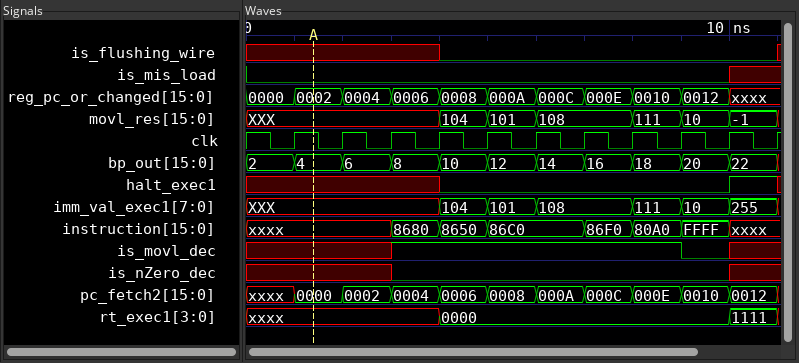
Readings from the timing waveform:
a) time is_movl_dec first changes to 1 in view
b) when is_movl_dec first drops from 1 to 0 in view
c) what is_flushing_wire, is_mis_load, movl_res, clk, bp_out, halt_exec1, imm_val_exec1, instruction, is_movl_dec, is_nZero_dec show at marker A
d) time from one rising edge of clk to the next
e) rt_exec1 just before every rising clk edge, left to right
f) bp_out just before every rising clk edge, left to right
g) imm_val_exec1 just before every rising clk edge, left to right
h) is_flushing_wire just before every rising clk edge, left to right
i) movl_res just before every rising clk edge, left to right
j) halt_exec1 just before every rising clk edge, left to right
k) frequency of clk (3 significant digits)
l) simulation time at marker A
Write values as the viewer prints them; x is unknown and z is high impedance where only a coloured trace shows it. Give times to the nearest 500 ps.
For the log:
3000 ps
9000 ps
is_flushing_wire=x, is_mis_load=0, movl_res=XXX, clk=1, bp_out=4, halt_exec1=x, imm_val_exec1=XXX, instruction=xxxx, is_movl_dec=x, is_nZero_dec=x
1000 ps
xxxx, xxxx, xxxx, xxxx, 0000, 0000, 0000, 0000, 0000, 0000, 1111
2, 4, 6, 8, 10, 12, 14, 16, 18, 20, 22
XXX, XXX, XXX, XXX, 104, 101, 108, 108, 111, 10, 255
x x x x 0 0 0 0 0 0 0
XXX, XXX, XXX, XXX, 104, 101, 108, 108, 111, 10, -1
x x x x 0 0 0 0 0 0 1
1.00 GHz
1500 ps
